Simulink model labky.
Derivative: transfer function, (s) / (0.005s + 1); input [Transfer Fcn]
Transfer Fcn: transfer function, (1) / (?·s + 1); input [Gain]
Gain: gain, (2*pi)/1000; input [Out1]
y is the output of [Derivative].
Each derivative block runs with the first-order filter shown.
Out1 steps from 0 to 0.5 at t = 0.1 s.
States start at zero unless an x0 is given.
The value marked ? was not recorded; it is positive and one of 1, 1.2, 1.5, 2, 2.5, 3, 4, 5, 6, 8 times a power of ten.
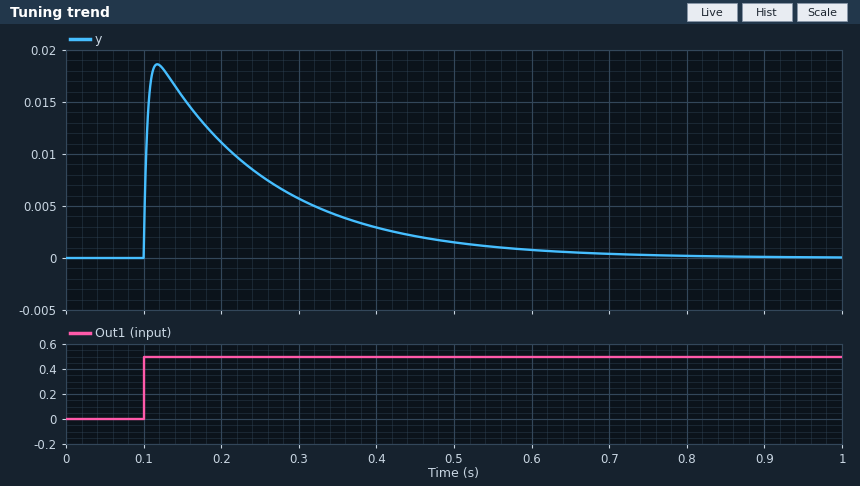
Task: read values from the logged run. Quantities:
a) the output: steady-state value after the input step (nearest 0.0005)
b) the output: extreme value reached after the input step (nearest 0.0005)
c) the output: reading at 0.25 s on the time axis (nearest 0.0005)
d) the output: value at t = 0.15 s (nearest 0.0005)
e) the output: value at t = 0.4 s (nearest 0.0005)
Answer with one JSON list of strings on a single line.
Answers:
["0.0000", "0.0185", "0.0080", "0.0155", "0.0030"]
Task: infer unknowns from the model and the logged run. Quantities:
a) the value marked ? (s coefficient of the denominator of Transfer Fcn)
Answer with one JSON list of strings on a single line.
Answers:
["0.15"]
